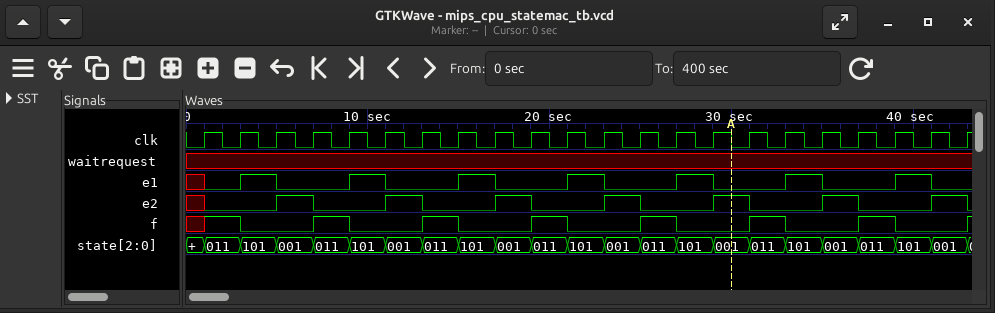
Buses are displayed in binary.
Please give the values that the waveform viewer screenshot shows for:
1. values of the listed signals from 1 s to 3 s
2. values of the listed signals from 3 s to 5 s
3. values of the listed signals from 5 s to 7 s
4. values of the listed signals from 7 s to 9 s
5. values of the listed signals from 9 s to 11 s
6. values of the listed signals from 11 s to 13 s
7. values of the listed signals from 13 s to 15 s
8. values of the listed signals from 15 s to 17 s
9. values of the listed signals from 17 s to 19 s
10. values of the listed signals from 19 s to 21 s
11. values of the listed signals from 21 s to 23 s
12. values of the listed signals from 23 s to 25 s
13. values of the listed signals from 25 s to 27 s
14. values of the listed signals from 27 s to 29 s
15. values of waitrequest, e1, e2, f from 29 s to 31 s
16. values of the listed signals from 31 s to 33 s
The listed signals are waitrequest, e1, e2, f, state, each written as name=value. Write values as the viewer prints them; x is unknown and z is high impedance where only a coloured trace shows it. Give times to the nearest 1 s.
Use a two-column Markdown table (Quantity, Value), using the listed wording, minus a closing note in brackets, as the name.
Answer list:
| Quantity | Value |
|---|---|
| values of the listed signals from 1 s to 3 s | waitrequest=x, e1=0, e2=0, f=1, state=011 |
| values of the listed signals from 3 s to 5 s | waitrequest=x, e1=1, e2=0, f=0, state=101 |
| values of the listed signals from 5 s to 7 s | waitrequest=x, e1=0, e2=1, f=0, state=001 |
| values of the listed signals from 7 s to 9 s | waitrequest=x, e1=0, e2=0, f=1, state=011 |
| values of the listed signals from 9 s to 11 s | waitrequest=x, e1=1, e2=0, f=0, state=101 |
| values of the listed signals from 11 s to 13 s | waitrequest=x, e1=0, e2=1, f=0, state=001 |
| values of the listed signals from 13 s to 15 s | waitrequest=x, e1=0, e2=0, f=1, state=011 |
| values of the listed signals from 15 s to 17 s | waitrequest=x, e1=1, e2=0, f=0, state=101 |
| values of the listed signals from 17 s to 19 s | waitrequest=x, e1=0, e2=1, f=0, state=001 |
| values of the listed signals from 19 s to 21 s | waitrequest=x, e1=0, e2=0, f=1, state=011 |
| values of the listed signals from 21 s to 23 s | waitrequest=x, e1=1, e2=0, f=0, state=101 |
| values of the listed signals from 23 s to 25 s | waitrequest=x, e1=0, e2=1, f=0, state=001 |
| values of the listed signals from 25 s to 27 s | waitrequest=x, e1=0, e2=0, f=1, state=011 |
| values of the listed signals from 27 s to 29 s | waitrequest=x, e1=1, e2=0, f=0, state=101 |
| values of waitrequest, e1, e2, f from 29 s to 31 s | waitrequest=x, e1=0, e2=1, f=0 |
| values of the listed signals from 31 s to 33 s | waitrequest=x, e1=0, e2=0, f=1, state=011 |
